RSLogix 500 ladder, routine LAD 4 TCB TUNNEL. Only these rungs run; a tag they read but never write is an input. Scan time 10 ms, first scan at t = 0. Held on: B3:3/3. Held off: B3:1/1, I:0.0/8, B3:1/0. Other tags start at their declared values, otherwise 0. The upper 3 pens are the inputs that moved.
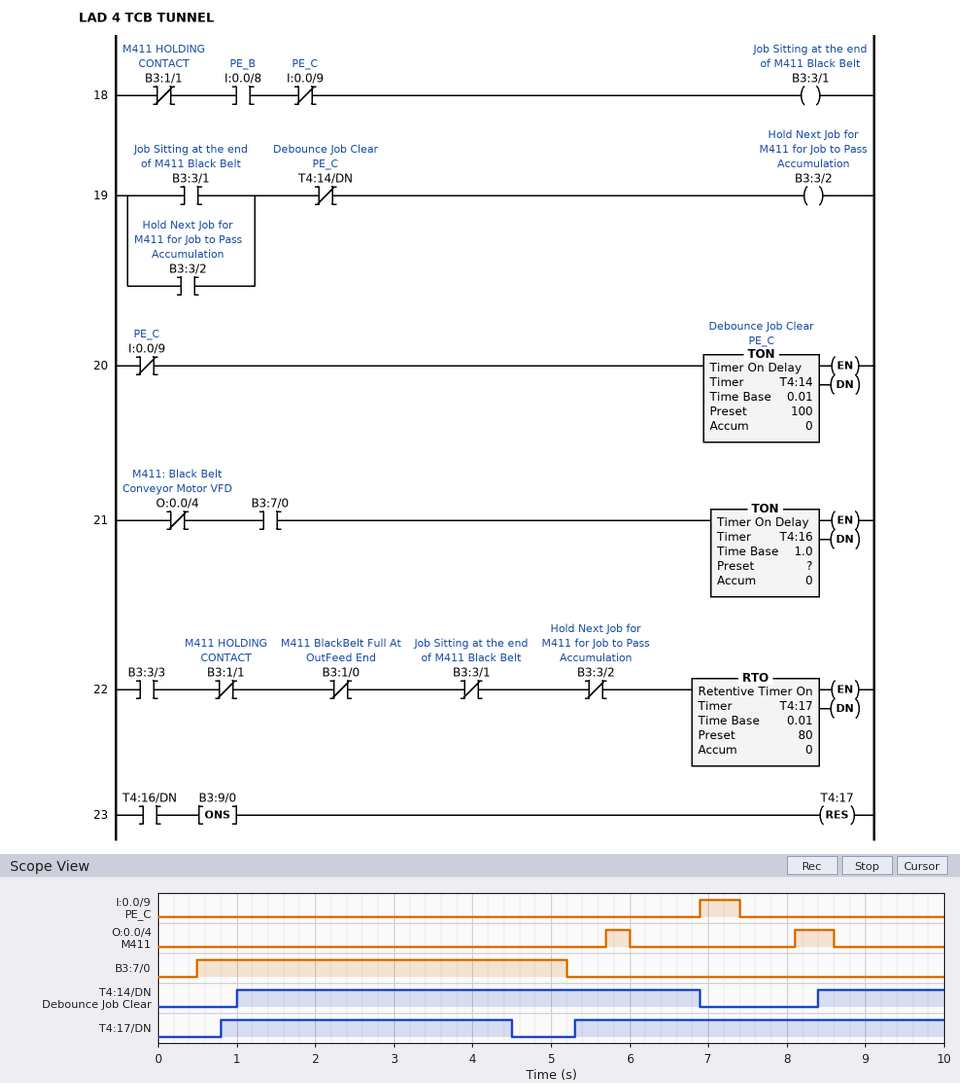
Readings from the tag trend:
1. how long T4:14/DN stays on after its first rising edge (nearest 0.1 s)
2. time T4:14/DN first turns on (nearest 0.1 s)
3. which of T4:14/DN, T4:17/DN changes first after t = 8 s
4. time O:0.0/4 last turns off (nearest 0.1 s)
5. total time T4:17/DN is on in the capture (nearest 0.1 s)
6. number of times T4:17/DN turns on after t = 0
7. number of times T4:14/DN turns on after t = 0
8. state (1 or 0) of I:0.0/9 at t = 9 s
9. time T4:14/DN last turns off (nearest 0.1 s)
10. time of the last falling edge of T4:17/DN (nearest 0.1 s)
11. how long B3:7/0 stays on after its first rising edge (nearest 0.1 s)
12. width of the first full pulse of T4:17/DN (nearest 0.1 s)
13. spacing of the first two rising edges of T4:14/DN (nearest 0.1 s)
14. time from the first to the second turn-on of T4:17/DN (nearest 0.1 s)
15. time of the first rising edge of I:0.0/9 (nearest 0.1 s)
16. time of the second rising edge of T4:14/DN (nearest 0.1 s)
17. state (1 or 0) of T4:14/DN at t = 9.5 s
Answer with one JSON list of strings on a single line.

["5.9 s", "1.0 s", "T4:14/DN", "8.6 s", "8.4 s", "2", "2", "0", "6.9 s", "4.5 s", "4.7 s", "3.7 s", "7.4 s", "4.5 s", "6.9 s", "8.4 s", "1"]
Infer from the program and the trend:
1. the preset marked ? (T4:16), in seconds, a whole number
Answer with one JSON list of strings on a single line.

["4 s"]
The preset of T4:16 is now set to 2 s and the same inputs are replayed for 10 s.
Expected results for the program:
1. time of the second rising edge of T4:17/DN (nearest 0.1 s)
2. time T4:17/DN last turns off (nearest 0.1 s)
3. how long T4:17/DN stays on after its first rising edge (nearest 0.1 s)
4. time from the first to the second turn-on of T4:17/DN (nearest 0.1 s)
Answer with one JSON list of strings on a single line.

["3.3 s", "2.5 s", "1.7 s", "2.5 s"]
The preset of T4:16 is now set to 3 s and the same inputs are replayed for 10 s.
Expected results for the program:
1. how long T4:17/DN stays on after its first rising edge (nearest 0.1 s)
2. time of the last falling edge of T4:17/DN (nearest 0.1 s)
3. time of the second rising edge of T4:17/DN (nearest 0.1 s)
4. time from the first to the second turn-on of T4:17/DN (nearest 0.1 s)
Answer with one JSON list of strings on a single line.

["2.7 s", "3.5 s", "4.3 s", "3.5 s"]
